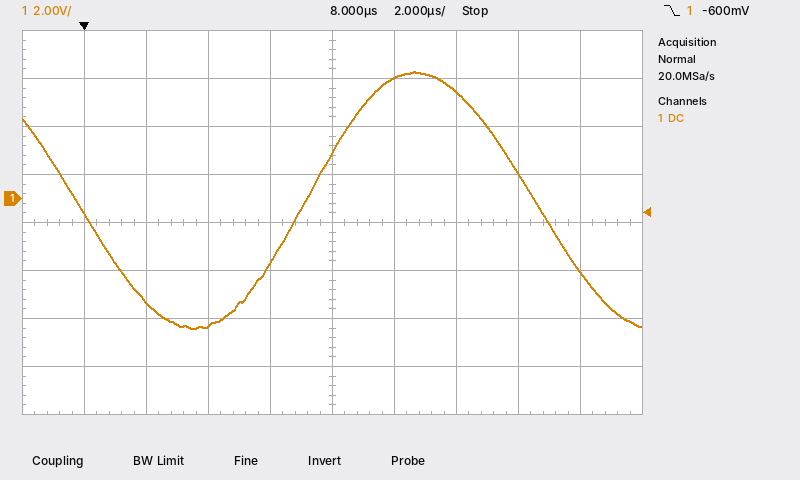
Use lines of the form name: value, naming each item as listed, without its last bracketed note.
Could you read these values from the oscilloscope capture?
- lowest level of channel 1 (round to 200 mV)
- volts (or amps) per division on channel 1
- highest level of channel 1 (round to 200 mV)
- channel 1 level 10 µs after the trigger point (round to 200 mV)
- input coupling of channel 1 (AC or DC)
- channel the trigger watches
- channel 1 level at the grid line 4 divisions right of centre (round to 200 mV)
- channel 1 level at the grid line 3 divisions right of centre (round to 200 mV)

lowest level of channel 1: -5.4 V
volts (or amps) per division on channel 1: 2 V
highest level of channel 1: 5.2 V
channel 1 level 10 µs after the trigger point: 5.0 V
input coupling of channel 1: DC
channel the trigger watches: channel 1
channel 1 level at the grid line 4 divisions right of centre: -3.0 V
channel 1 level at the grid line 3 divisions right of centre: 1.0 V
